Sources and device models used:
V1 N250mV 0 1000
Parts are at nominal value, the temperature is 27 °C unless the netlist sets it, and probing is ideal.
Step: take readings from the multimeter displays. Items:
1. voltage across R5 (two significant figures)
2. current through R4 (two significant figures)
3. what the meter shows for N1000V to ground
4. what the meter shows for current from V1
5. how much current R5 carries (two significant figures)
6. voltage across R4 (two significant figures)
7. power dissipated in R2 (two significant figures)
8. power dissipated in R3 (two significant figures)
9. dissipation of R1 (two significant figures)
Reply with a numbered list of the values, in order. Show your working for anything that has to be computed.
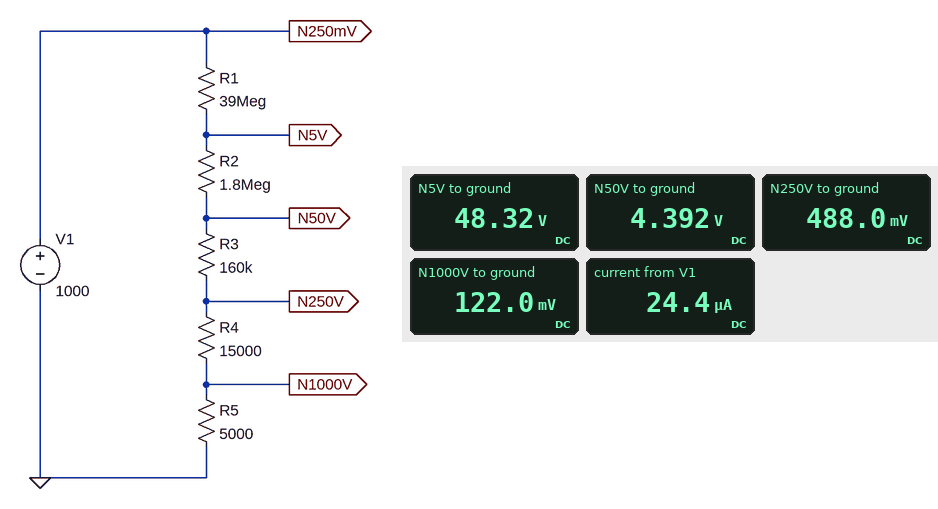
1. 122 mV = 120 mV
2. (488 mV - 122 mV) / 15 kΩ = 24 µA
3. 122.0 mV
4. 24.4 µA
5. (122 mV) / 5 kΩ = 24 µA
6. 488 mV - 122 mV = 370 mV
7. (48.32 V - 4.392 V)^2 / 1.8 MΩ = 1.1 mW
8. (4.392 V - 488 mV)^2 / 160 kΩ = 95 µW
9. (1 kV - 48.32 V)^2 / 39 MΩ = 23 mW
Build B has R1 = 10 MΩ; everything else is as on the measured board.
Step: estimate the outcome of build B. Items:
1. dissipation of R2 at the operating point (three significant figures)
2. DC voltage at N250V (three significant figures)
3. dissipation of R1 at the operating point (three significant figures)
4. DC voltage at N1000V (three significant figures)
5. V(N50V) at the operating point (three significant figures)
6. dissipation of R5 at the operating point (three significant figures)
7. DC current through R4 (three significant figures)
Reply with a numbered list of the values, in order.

1. 12.5 mW
2. 1.67 V
3. 69.7 mW
4. 417 mV
5. 15.0 V
6. 34.8 µW
7. 83.5 µA
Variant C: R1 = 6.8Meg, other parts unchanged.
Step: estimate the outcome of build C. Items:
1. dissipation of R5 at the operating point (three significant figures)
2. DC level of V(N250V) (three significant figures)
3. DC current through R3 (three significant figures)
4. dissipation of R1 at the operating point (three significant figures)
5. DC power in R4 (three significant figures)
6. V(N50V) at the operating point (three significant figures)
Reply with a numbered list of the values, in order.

1. 64.9 µW
2. 2.28 V
3. 114 µA
4. 88.2 mW
5. 195 µW
6. 20.5 V
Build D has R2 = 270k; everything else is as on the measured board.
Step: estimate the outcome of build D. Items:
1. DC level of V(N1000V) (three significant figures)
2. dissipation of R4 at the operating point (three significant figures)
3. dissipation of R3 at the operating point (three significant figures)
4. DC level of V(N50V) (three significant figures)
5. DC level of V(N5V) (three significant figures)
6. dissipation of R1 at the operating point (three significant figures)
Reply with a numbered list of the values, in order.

1. 127 mV
2. 9.64 µW
3. 103 µW
4. 4.56 V
5. 11.4 V
6. 25.1 mW
